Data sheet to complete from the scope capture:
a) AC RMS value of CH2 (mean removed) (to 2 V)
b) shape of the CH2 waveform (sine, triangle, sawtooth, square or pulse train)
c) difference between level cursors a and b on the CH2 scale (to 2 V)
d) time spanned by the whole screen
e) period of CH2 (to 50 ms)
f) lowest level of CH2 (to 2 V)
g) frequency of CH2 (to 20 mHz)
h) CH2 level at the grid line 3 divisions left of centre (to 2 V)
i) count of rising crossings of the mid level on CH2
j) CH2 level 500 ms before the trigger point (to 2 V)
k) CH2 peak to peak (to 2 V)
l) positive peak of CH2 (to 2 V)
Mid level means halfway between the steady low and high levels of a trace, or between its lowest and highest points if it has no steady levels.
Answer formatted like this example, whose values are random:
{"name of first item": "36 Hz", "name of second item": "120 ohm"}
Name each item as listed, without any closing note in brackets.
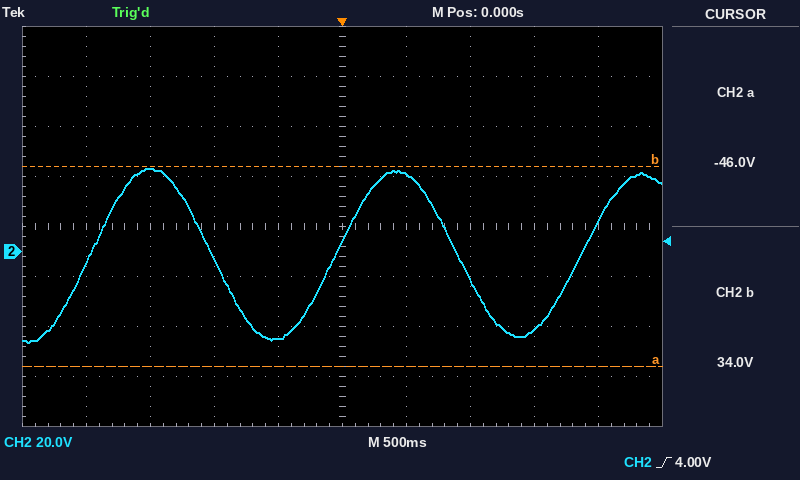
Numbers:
{"AC RMS value of CH2 (mean removed)": "24 V", "shape of the CH2 waveform": "sine", "difference between level cursors a and b on the CH2 scale": "80 V", "time spanned by the whole screen": "5 s", "period of CH2": "1.90 s", "lowest level of CH2": "-36 V", "frequency of CH2": "520 mHz", "CH2 level at the grid line 3 divisions left of centre": "34 V", "count of rising crossings of the mid level on CH2": "3", "CH2 level 500 ms before the trigger point": "-34 V", "CH2 peak to peak": "70 V", "positive peak of CH2": "34 V"}
